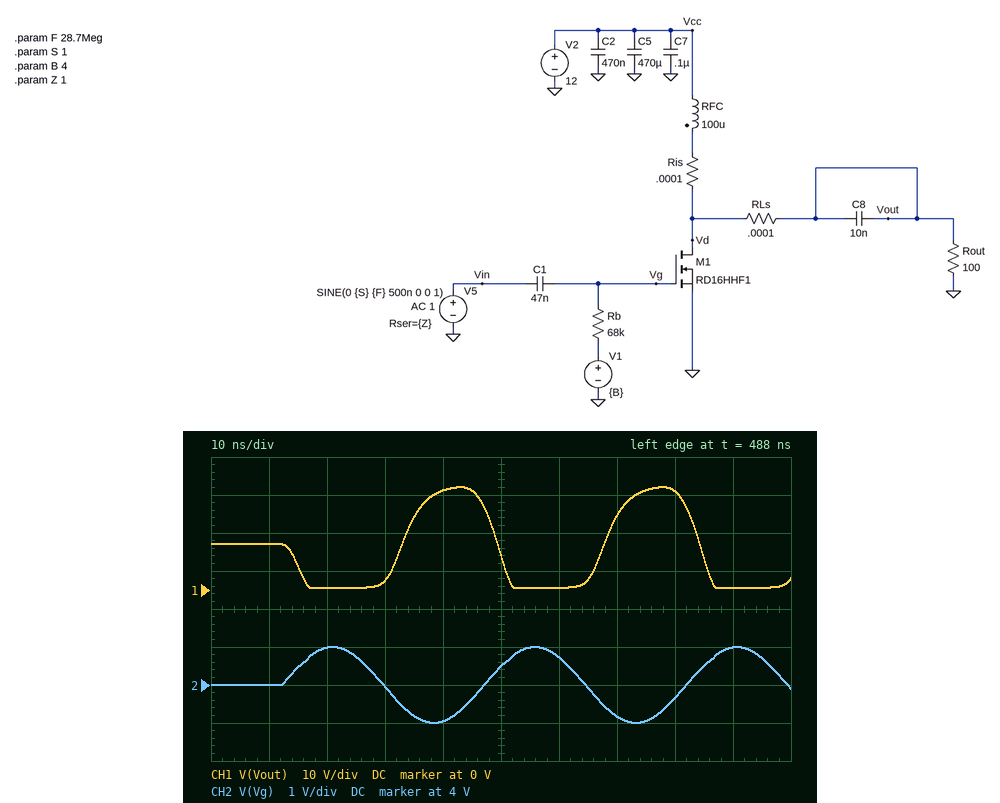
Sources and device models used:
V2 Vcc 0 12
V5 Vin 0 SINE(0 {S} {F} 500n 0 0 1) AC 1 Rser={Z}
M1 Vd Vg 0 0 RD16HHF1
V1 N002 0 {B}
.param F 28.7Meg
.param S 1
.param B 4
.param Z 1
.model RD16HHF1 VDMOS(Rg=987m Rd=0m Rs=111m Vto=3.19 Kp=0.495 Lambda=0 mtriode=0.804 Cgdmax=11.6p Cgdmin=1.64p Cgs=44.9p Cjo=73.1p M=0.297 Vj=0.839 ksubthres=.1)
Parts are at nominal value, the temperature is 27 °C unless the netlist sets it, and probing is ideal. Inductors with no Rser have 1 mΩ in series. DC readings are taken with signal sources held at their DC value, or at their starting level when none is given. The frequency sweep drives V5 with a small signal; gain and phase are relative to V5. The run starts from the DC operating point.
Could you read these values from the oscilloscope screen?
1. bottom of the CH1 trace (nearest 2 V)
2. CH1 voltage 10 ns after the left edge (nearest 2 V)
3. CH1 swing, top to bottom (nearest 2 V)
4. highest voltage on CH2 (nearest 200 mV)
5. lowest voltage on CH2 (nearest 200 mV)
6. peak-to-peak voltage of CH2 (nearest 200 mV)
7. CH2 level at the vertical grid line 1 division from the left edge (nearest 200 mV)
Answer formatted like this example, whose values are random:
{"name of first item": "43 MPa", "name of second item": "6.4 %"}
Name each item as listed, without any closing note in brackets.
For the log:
{"bottom of the CH1 trace": "0 V", "CH1 voltage 10 ns after the left edge": "12 V", "CH1 swing, top to bottom": "26 V", "highest voltage on CH2": "5.0 V", "lowest voltage on CH2": "3.0 V", "peak-to-peak voltage of CH2": "2.0 V", "CH2 level at the vertical grid line 1 division from the left edge": "4.0 V"}
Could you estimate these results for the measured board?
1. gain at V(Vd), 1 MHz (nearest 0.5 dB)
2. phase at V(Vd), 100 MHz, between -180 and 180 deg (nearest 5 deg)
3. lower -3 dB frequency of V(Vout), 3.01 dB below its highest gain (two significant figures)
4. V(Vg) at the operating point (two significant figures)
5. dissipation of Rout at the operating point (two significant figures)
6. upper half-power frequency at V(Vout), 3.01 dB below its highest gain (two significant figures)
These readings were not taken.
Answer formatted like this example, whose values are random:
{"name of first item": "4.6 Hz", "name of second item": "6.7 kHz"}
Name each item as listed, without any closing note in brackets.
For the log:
{"gain at V(Vd), 1 MHz": "31.5 dB", "phase at V(Vd), 100 MHz, between -180 and 180 deg": "110 deg", "lower -3 dB frequency of V(Vout), 3.01 dB below its highest gain": "160 kHz", "V(Vg) at the operating point": "4.0 V", "dissipation of Rout at the operating point": "1.4 W", "upper half-power frequency at V(Vout), 3.01 dB below its highest gain": "44 MHz"}
